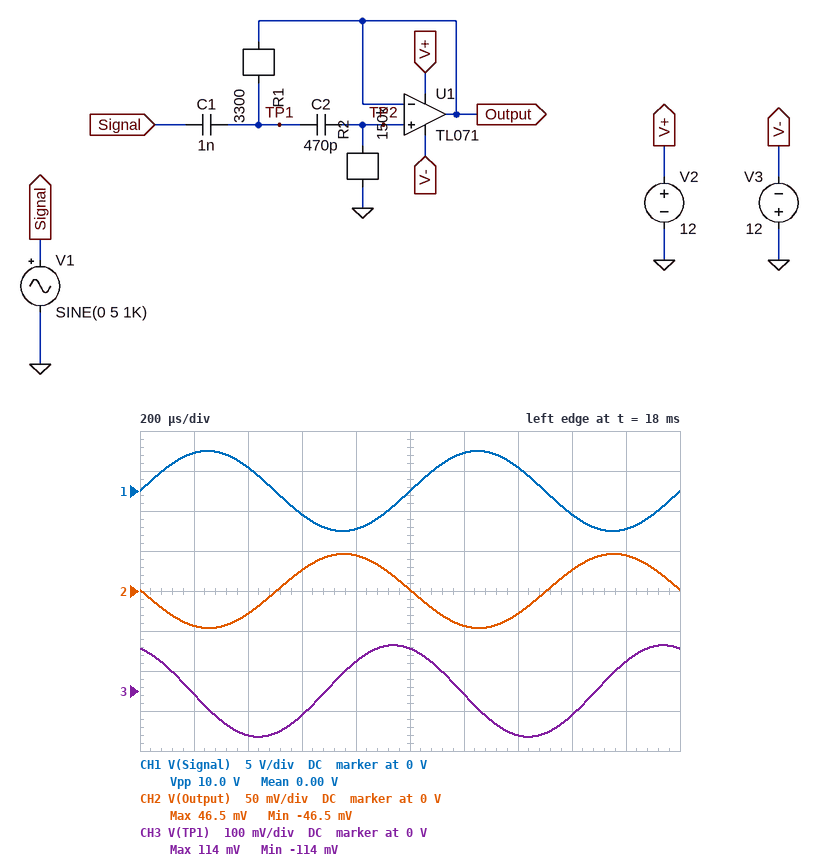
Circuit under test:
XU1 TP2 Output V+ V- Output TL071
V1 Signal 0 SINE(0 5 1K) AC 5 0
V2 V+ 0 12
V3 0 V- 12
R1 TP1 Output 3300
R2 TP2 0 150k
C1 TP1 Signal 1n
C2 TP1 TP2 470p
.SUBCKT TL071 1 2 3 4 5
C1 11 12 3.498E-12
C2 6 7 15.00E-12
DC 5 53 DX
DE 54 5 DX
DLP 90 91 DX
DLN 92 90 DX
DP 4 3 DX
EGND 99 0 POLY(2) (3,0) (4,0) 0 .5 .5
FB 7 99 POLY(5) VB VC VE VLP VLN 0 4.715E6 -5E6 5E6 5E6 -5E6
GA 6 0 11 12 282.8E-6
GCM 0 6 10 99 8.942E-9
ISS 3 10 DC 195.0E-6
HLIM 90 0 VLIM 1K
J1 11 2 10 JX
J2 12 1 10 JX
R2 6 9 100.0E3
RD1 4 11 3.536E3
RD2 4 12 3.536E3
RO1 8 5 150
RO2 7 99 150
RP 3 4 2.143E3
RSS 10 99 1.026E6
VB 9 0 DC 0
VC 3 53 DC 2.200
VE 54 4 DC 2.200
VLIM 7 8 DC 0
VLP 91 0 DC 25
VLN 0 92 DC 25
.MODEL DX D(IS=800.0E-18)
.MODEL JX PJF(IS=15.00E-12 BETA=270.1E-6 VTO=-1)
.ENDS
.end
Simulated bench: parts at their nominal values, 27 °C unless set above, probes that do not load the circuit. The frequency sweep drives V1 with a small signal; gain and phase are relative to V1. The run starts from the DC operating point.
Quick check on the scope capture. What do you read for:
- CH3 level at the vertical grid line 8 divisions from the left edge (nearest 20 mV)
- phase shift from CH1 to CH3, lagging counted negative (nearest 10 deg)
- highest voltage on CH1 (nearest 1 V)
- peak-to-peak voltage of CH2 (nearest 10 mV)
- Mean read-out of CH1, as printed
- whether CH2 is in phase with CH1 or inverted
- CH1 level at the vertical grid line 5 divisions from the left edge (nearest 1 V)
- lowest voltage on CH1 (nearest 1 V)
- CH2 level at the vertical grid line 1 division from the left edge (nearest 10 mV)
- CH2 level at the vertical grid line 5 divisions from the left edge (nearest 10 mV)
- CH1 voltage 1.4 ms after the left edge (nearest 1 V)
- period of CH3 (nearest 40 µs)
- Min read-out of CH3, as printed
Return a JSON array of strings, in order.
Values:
["-60 mV", "110 deg", "5 V", "90 mV", "0.00 V", "inverted", "0 V", "-5 V", "-40 mV", "0 V", "3 V", "1.00 ms", "-114 mV"]
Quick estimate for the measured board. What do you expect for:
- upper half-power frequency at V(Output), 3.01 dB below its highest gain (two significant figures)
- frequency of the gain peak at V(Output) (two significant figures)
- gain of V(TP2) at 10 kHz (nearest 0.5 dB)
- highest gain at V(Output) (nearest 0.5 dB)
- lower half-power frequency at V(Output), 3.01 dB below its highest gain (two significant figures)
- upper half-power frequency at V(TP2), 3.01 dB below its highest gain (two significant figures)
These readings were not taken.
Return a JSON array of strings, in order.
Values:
["13 kHz", "11 kHz", "9.5 dB", "10.0 dB", "9.2 kHz", "13 kHz"]
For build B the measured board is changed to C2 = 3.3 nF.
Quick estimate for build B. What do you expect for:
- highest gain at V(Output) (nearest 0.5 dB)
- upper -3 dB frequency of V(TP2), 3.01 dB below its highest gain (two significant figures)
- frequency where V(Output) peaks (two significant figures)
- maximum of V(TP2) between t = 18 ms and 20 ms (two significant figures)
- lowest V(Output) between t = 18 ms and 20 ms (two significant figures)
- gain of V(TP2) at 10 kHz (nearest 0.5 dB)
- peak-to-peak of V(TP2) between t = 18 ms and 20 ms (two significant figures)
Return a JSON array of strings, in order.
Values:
["9.0 dB", "5.1 kHz", "4.0 kHz", "340 mV", "-340 mV", "1.0 dB", "690 mV"]
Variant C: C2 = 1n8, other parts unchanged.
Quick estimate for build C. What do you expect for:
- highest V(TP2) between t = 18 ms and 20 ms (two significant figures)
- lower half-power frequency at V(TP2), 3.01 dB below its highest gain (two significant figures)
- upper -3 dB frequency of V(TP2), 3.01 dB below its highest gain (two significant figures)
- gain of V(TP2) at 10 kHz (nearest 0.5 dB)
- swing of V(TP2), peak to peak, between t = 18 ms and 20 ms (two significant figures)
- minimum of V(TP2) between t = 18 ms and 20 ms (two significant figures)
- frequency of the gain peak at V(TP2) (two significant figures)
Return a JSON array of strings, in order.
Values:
["180 mV", "4.7 kHz", "6.6 kHz", "2.5 dB", "360 mV", "-180 mV", "5.4 kHz"]
